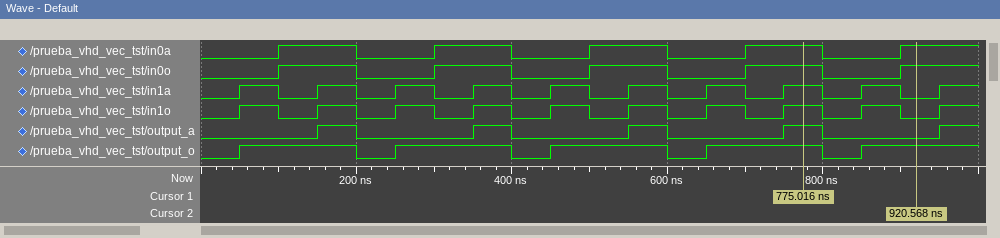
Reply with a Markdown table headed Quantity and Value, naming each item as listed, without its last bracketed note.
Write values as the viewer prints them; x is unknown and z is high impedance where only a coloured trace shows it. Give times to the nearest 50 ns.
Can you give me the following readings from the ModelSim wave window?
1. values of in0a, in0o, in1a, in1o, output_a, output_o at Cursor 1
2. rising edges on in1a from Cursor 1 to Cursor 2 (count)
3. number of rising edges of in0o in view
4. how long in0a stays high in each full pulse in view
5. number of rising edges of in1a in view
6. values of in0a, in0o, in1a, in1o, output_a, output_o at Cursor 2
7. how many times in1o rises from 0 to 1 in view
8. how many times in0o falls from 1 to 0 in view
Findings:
| Quantity | Value |
|---|---|
| values of in0a, in0o, in1a, in1o, output_a, output_o at Cursor 1 | in0a=1, in0o=1, in1a=1, in1o=1, output_a=1, output_o=1 |
| rising edges on in1a from Cursor 1 to Cursor 2 | 1 |
| number of rising edges of in0o in view | 5 |
| how long in0a stays high in each full pulse in view | 100 ns, 100 ns, 100 ns, 100 ns |
| number of rising edges of in1a in view | 10 |
| values of in0a, in0o, in1a, in1o, output_a, output_o at Cursor 2 | in0a=1, in0o=1, in1a=0, in1o=0, output_a=0, output_o=1 |
| how many times in1o rises from 0 to 1 in view | 10 |
| how many times in0o falls from 1 to 0 in view | 4 |
